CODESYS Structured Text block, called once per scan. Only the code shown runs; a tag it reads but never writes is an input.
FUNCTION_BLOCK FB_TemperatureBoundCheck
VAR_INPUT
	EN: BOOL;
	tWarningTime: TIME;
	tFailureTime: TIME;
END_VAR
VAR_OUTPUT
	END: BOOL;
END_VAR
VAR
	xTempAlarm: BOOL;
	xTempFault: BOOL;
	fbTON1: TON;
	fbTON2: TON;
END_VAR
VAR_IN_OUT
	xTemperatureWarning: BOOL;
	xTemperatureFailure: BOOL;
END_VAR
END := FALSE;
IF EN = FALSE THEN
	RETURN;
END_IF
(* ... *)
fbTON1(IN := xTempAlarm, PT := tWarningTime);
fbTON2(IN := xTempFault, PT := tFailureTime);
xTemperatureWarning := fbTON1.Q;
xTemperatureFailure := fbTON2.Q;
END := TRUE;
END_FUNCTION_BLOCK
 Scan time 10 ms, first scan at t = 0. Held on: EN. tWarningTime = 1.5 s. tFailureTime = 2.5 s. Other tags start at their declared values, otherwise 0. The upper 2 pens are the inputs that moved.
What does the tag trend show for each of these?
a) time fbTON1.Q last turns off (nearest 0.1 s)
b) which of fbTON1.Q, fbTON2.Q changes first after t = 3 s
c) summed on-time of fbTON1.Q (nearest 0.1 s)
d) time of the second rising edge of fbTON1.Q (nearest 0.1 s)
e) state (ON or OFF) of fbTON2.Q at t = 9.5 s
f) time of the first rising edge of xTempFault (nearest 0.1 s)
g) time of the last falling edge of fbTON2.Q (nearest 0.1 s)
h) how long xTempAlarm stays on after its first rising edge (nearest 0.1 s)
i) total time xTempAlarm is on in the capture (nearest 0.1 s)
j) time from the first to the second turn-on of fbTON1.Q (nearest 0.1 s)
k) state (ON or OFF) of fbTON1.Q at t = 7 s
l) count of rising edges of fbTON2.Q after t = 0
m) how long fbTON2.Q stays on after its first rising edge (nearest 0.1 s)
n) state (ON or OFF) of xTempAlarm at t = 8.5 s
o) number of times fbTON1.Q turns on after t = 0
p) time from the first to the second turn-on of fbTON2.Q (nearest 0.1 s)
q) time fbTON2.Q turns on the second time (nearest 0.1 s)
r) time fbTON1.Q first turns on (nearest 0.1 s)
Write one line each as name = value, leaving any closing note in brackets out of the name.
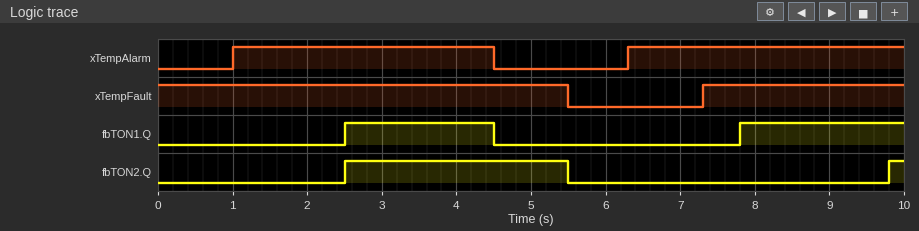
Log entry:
time fbTON1.Q last turns off = 4.5 s
which of fbTON1.Q, fbTON2.Q changes first after t = 3 s = fbTON1.Q
summed on-time of fbTON1.Q = 4.2 s
time of the second rising edge of fbTON1.Q = 7.8 s
state (ON or OFF) of fbTON2.Q at t = 9.5 s = OFF
time of the first rising edge of xTempFault = 7.3 s
time of the last falling edge of fbTON2.Q = 5.5 s
how long xTempAlarm stays on after its first rising edge = 3.5 s
total time xTempAlarm is on in the capture = 7.2 s
time from the first to the second turn-on of fbTON1.Q = 5.3 s
state (ON or OFF) of fbTON1.Q at t = 7 s = OFF
count of rising edges of fbTON2.Q after t = 0 = 2
how long fbTON2.Q stays on after its first rising edge = 3.0 s
state (ON or OFF) of xTempAlarm at t = 8.5 s = ON
number of times fbTON1.Q turns on after t = 0 = 2
time from the first to the second turn-on of fbTON2.Q = 7.3 s
time fbTON2.Q turns on the second time = 9.8 s
time fbTON1.Q first turns on = 2.5 s
